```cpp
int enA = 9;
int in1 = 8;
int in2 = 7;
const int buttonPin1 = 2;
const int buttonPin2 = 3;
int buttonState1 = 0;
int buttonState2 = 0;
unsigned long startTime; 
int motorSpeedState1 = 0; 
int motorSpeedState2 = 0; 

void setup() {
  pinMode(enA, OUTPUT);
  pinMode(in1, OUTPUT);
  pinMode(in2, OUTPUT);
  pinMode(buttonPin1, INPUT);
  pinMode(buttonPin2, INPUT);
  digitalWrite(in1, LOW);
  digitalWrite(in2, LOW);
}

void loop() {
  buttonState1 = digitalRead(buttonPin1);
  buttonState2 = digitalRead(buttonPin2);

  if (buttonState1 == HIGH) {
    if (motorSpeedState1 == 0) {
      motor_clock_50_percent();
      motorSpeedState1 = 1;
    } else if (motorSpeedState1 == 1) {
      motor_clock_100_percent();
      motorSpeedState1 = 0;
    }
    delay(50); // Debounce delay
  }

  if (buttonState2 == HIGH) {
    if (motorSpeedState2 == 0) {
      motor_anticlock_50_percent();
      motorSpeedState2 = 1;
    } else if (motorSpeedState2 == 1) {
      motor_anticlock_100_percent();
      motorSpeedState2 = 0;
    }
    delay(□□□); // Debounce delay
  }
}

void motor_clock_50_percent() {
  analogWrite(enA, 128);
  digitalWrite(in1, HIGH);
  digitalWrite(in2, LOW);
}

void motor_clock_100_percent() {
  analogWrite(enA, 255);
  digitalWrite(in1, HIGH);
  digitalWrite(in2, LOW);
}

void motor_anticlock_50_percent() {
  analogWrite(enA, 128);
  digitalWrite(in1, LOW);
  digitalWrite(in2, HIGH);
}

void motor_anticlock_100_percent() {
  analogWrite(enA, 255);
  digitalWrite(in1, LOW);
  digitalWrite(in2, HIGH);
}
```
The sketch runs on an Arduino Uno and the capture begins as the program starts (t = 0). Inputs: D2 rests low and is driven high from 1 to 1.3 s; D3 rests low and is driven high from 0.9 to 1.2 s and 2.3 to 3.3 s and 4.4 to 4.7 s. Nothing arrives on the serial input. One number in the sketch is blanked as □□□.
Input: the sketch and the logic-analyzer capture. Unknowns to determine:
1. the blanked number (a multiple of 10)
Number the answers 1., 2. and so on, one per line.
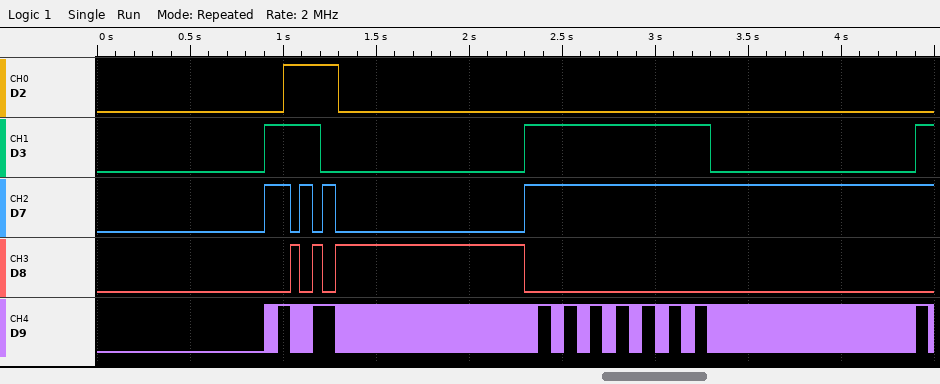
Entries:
1. 70
